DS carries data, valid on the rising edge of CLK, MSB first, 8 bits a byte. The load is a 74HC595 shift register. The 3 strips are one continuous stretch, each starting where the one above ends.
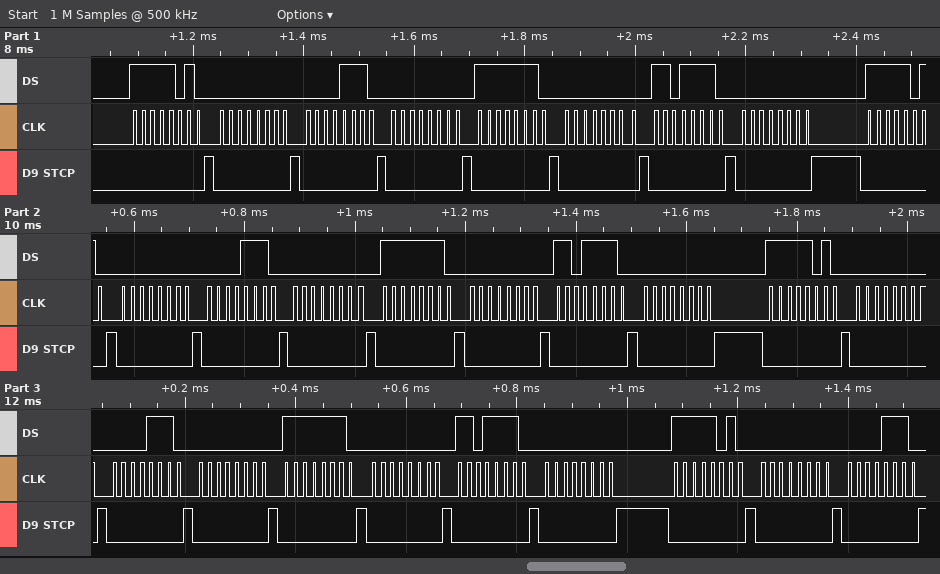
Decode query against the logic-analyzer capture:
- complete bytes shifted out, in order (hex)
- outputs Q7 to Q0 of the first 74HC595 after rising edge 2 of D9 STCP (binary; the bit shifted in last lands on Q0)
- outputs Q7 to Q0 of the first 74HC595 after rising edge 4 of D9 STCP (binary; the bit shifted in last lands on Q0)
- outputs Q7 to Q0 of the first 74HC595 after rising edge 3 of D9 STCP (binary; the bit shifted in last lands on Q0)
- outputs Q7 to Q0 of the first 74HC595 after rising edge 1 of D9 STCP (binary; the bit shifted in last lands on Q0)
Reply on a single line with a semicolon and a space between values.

0xFA 0x00 0x0E 0x00 0xFE 0x00 0xDE 0x00 0xFA 0x00 0x0E 0x00 0xFE 0x00 0xDE 0x00 0xFA 0x00 0x0E 0x00 0xFE 0x00 0xDE 0x00 0xFA 0x00 0x0E; 00000000; 00000000; 00001110; 11111010
